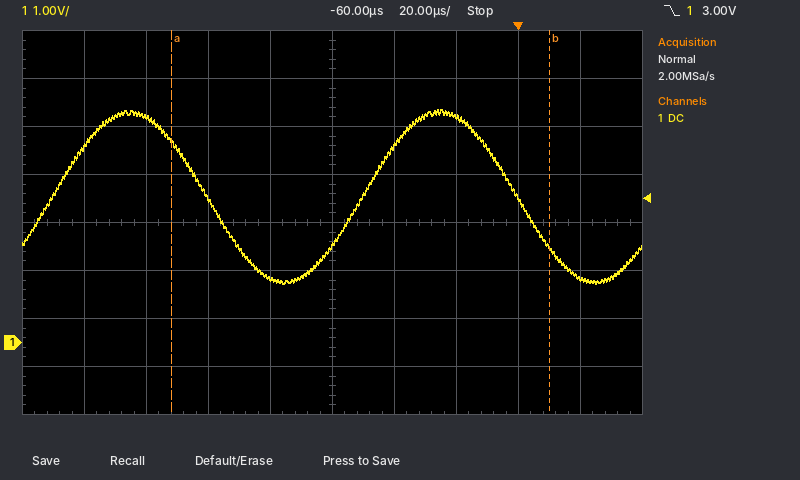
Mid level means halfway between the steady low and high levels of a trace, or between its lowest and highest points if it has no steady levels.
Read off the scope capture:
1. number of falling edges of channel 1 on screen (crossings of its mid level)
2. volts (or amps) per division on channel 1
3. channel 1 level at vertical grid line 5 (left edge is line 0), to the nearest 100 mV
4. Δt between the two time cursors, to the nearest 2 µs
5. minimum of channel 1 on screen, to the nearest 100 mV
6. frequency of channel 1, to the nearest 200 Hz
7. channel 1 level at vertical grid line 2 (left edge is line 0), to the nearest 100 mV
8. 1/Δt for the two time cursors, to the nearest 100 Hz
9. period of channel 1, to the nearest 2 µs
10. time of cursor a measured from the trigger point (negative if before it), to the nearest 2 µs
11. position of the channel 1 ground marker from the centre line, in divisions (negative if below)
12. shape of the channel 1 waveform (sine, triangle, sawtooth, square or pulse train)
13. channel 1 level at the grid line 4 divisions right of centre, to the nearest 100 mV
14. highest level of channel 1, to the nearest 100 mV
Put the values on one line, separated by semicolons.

2; 1 V; 2.0 V; 122 µs; 1.2 V; 10.0 kHz; 4.7 V; 8.2 kHz; 100 µs; -112 µs; -2.5 div; sine; 1.3 V; 4.9 V
